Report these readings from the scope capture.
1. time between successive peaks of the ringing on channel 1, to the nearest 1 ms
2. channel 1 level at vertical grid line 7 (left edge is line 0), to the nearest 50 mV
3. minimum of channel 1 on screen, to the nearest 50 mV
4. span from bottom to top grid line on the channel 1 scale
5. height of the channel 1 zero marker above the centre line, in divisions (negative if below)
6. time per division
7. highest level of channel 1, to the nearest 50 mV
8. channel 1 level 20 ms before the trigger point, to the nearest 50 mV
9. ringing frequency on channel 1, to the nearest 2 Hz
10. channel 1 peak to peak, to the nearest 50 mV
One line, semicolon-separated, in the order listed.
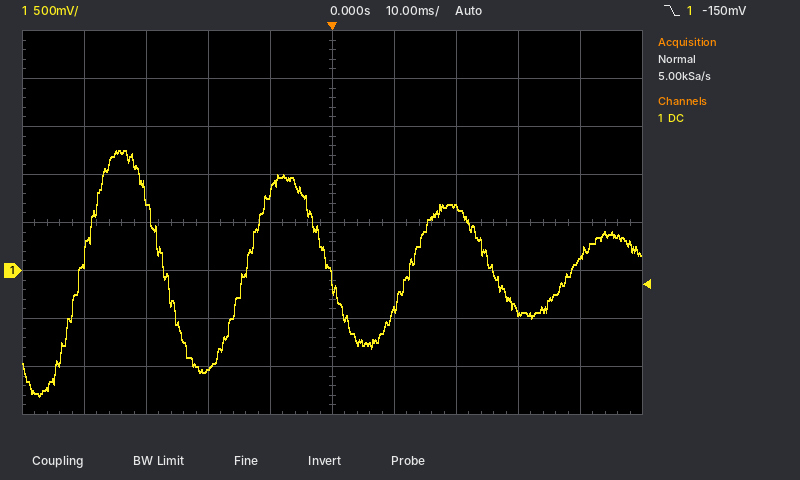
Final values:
26 ms; 650 mV; -1.30 V; 4 V; -1.0 div; 10 ms; 1.25 V; -1.05 V; 38 Hz; 2.55 V
